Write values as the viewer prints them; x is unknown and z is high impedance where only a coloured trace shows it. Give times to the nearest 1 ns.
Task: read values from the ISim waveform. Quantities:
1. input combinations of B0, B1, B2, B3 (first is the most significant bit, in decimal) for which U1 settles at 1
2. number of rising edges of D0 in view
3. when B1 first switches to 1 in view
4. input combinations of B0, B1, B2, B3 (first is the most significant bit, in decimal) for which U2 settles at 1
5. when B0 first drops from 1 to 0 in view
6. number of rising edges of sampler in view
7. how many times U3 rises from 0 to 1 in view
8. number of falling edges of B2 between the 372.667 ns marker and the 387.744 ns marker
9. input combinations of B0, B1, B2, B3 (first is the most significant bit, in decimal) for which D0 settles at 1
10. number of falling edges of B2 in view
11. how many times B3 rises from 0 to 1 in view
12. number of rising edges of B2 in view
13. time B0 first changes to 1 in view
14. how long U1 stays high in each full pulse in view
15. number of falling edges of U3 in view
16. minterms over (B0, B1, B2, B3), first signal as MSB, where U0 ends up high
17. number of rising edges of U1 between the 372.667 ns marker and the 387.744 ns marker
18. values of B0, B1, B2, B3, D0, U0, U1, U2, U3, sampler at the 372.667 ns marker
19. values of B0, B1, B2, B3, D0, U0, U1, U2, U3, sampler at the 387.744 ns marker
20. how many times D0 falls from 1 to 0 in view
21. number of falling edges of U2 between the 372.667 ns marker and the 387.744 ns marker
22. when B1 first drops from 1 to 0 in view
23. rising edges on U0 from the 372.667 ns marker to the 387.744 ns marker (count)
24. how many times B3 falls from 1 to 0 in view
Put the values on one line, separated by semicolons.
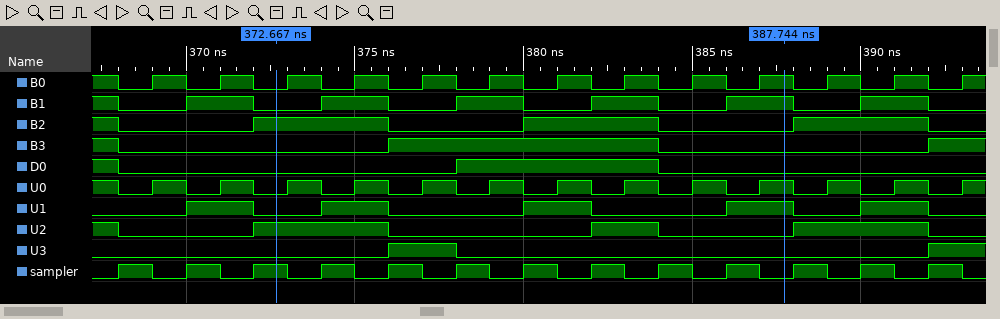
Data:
3, 4, 6, 11, 12, 14; 1; 370 ns; 2, 6, 7, 10, 14, 15; 368 ns; 13; 2; 2; 3, 5, 7, 11, 13, 15; 4; 2; 3; 369 ns; 2 ns, 2 ns, 2 ns, 2 ns, 2 ns; 1; 8, 9, 10, 11, 12, 13, 14, 15; 3; B0=0, B1=0, B2=1, B3=0, D0=0, U0=0, U1=0, U2=1, U3=0, sampler=1; B0=1, B1=1, B2=0, B3=0, D0=0, U0=1, U1=1, U2=0, U3=0, sampler=0; 2; 2; 368 ns; 8; 2
